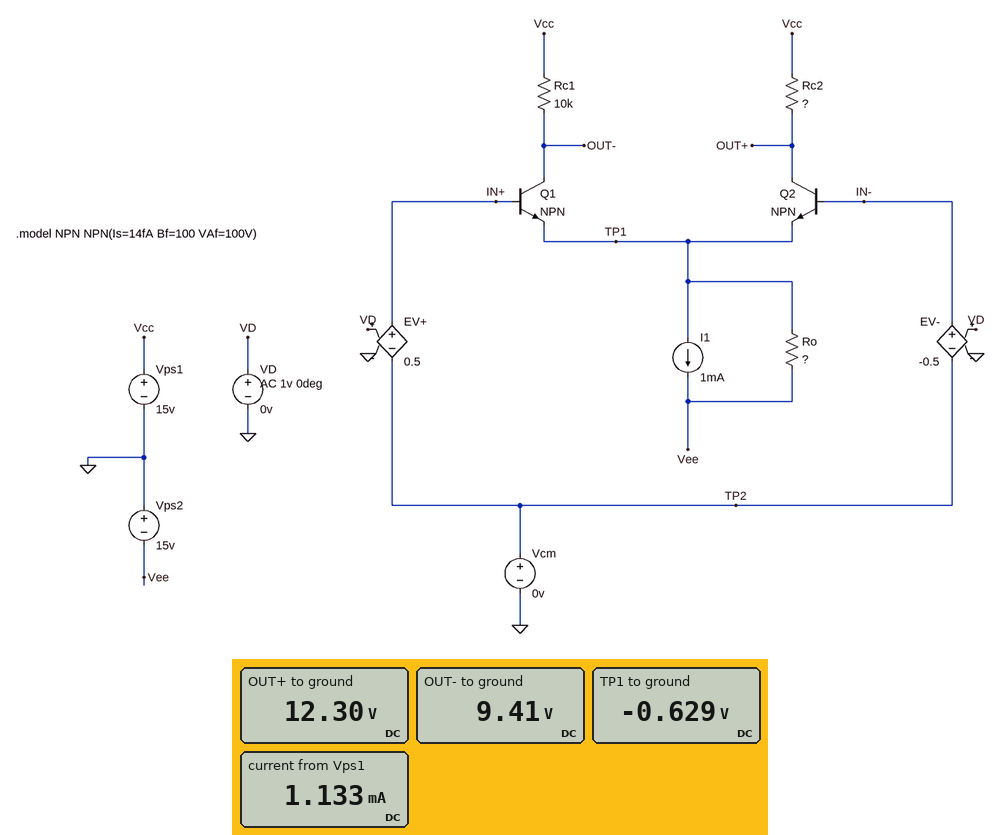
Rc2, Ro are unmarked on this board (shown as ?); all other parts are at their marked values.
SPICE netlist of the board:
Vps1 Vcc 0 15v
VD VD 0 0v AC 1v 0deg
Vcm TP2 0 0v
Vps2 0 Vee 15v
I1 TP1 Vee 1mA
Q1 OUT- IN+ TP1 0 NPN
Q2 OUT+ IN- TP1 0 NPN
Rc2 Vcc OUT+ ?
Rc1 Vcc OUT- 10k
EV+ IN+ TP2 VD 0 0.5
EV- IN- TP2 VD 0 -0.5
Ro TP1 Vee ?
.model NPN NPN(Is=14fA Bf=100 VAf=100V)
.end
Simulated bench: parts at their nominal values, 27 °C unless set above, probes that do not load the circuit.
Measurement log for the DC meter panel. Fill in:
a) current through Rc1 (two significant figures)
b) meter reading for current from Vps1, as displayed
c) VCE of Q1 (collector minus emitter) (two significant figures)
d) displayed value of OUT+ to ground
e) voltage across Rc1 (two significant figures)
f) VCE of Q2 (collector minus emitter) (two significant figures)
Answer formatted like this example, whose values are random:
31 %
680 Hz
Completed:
560 µA
1.133 mA
10 V
12.30 V
5.6 V
13 V
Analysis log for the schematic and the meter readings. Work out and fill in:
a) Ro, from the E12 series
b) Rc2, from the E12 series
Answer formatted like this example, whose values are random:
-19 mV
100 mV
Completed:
100 kΩ
4.7 kΩ
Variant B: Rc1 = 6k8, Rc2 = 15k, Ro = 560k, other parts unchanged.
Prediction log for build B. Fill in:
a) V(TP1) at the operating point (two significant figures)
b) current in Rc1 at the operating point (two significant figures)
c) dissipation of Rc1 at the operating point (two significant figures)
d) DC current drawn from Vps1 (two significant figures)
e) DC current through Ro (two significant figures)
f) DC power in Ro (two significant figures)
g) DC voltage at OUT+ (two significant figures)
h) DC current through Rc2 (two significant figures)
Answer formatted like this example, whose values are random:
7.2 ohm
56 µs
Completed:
-630 mV
520 µA
1.8 mW
1.0 mA
26 µA
370 µW
7.5 V
500 µA
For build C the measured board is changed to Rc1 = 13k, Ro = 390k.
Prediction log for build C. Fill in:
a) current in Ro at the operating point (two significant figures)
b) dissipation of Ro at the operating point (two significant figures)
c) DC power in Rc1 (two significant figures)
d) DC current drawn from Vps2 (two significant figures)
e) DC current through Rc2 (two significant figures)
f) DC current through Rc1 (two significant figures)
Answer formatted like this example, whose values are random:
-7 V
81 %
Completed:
37 µA
530 µW
3.3 mW
1.0 mA
520 µA
500 µA
